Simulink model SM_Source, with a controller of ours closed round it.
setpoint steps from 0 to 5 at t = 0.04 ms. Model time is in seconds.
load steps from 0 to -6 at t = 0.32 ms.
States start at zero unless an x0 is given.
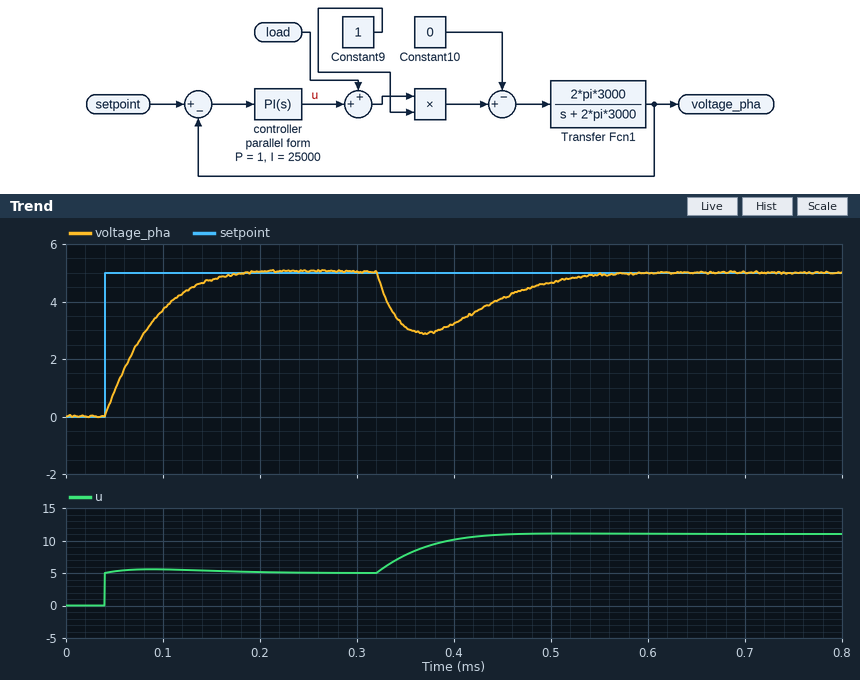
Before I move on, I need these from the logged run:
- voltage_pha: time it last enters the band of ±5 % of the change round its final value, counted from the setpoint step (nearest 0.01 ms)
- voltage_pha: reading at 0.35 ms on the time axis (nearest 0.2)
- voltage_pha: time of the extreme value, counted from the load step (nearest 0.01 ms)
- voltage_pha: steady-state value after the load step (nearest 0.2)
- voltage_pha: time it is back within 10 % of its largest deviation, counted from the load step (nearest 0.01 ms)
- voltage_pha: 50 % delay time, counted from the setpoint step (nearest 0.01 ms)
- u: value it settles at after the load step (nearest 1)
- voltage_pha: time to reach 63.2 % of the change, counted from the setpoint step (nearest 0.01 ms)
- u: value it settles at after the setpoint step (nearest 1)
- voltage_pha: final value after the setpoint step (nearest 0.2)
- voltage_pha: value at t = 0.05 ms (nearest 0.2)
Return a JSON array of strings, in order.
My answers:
["0.11 ms", "3.2", "0.05 ms", "5.0", "0.20 ms", "0.03 ms", "11", "0.05 ms", "5", "5.0", "0.8"]
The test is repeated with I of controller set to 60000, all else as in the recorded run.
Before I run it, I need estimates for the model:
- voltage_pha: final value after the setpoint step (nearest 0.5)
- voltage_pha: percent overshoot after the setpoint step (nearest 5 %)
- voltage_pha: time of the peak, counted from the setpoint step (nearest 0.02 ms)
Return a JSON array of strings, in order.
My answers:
["5.0", "15 %", "0.10 ms"]
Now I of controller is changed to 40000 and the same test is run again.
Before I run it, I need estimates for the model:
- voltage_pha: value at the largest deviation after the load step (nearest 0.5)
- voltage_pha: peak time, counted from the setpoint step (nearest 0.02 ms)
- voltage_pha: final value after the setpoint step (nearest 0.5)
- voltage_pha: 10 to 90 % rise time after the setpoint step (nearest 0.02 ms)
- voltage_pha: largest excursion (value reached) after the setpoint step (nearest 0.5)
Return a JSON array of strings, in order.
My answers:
["3.0", "0.12 ms", "5.0", "0.06 ms", "5.5"]
